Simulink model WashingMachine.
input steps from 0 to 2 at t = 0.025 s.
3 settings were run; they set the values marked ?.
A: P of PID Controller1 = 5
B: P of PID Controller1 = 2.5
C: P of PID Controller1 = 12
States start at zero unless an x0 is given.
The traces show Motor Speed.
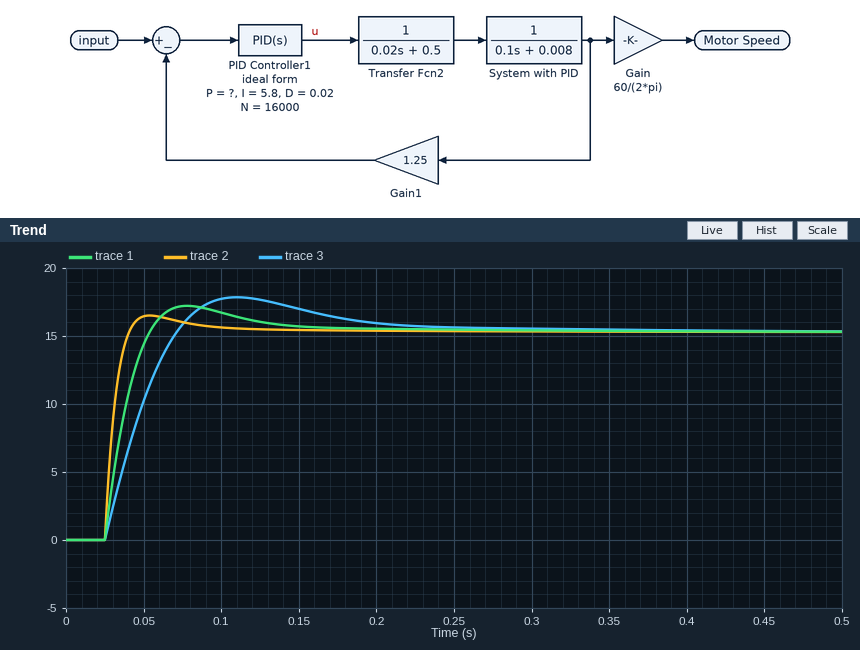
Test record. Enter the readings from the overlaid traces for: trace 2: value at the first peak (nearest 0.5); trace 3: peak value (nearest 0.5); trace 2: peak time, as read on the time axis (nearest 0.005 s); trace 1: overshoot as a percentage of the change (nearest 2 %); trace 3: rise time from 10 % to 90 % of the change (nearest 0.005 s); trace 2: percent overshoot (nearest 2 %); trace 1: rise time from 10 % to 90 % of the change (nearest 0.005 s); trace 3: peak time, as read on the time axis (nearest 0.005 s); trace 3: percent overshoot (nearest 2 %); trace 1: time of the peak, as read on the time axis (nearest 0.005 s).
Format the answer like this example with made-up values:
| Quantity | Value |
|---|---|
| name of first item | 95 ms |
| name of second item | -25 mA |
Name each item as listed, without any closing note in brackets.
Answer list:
| Quantity | Value |
|---|---|
| trace 2: value at the first peak | 16.5 |
| trace 3: peak value | 18.0 |
| trace 2: peak time, as read on the time axis | 0.055 s |
| trace 1: overshoot as a percentage of the change | 12 % |
| trace 3: rise time from 10 % to 90 % of the change | 0.035 s |
| trace 2: percent overshoot | 8 % |
| trace 1: rise time from 10 % to 90 % of the change | 0.020 s |
| trace 3: peak time, as read on the time axis | 0.110 s |
| trace 3: percent overshoot | 16 % |
| trace 1: time of the peak, as read on the time axis | 0.080 s |
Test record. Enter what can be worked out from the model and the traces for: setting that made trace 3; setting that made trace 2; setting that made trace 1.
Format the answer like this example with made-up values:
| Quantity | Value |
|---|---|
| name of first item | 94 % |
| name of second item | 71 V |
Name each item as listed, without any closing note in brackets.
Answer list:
| Quantity | Value |
|---|---|
| setting that made trace 3 | B |
| setting that made trace 2 | C |
| setting that made trace 1 | A |
